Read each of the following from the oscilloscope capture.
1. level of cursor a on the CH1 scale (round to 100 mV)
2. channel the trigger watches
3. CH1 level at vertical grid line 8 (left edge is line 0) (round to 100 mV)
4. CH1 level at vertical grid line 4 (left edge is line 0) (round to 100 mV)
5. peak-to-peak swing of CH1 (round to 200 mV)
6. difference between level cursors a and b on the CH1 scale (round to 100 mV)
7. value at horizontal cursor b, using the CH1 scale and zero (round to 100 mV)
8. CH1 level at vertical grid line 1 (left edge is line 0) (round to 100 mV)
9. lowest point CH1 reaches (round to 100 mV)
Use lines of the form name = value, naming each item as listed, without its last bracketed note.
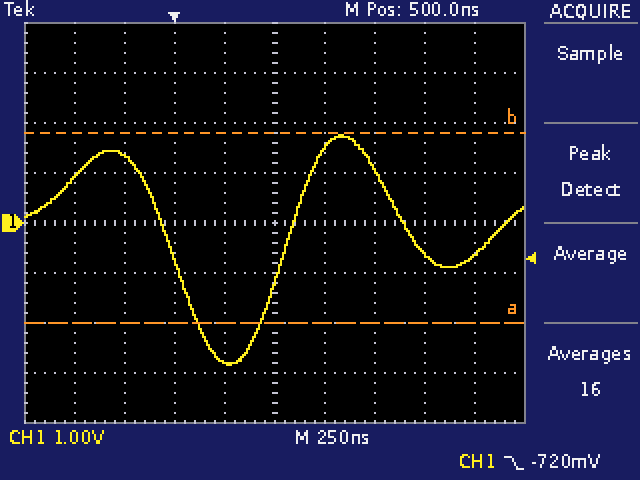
level of cursor a on the CH1 scale = -2.0 V
channel the trigger watches = CH1
CH1 level at vertical grid line 8 (left edge is line 0) = -600 mV
CH1 level at vertical grid line 4 (left edge is line 0) = -2.8 V
peak-to-peak swing of CH1 = 4.6 V
difference between level cursors a and b on the CH1 scale = 3.8 V
value at horizontal cursor b, using the CH1 scale and zero = 1.8 V
CH1 level at vertical grid line 1 (left edge is line 0) = 900 mV
lowest point CH1 reaches = -2.8 V
